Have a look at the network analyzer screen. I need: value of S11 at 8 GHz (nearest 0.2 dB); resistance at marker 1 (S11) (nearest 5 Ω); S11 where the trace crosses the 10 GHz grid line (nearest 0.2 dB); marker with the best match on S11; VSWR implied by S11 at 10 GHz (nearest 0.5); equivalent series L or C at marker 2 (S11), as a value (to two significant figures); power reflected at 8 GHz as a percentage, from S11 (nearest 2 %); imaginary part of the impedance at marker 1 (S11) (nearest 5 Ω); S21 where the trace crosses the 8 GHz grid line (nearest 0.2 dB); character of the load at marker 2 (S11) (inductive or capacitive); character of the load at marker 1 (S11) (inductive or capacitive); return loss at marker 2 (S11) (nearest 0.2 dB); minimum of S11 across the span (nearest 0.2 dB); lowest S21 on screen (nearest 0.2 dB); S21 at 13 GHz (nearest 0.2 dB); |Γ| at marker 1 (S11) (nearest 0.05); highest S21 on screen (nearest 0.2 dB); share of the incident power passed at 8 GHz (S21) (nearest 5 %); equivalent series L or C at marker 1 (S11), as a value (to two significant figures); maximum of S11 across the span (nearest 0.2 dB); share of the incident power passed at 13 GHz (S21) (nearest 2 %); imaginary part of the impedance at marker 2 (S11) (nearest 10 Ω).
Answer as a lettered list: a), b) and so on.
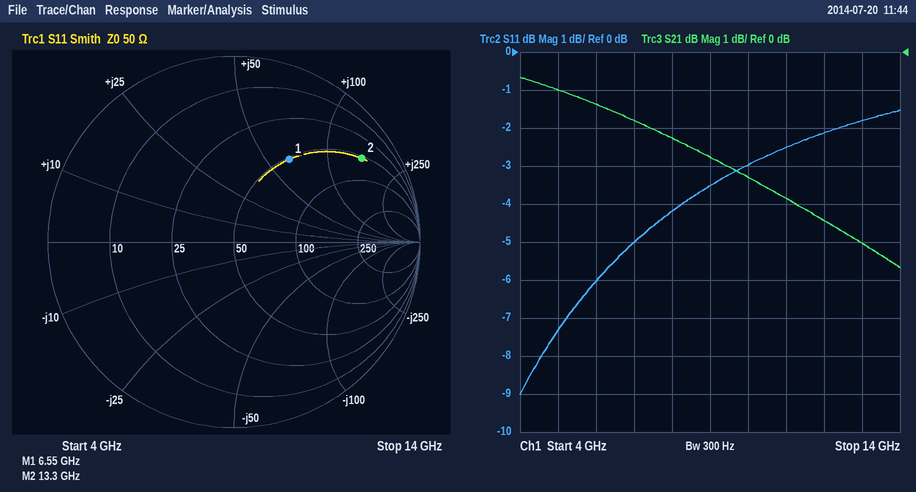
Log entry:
a) -4.2 dB
b) 50 Ω
c) -3.0 dB
d) marker 1
e) 6.0
f) 1.8 nH
g) 38 %
h) +65 Ω
i) -2.2 dB
j) inductive
k) inductive
l) 1.8 dB
m) -9.0 dB
n) -5.6 dB
o) -5.0 dB
p) 0.55
q) -0.6 dB
r) 60 %
s) 1.6 nH
t) -1.6 dB
u) 32 %
v) +150 Ω
